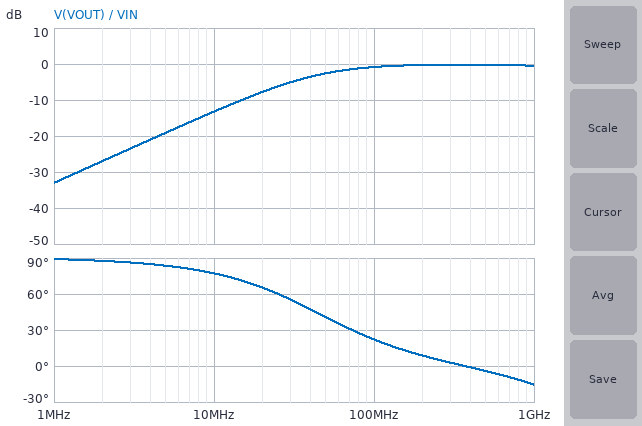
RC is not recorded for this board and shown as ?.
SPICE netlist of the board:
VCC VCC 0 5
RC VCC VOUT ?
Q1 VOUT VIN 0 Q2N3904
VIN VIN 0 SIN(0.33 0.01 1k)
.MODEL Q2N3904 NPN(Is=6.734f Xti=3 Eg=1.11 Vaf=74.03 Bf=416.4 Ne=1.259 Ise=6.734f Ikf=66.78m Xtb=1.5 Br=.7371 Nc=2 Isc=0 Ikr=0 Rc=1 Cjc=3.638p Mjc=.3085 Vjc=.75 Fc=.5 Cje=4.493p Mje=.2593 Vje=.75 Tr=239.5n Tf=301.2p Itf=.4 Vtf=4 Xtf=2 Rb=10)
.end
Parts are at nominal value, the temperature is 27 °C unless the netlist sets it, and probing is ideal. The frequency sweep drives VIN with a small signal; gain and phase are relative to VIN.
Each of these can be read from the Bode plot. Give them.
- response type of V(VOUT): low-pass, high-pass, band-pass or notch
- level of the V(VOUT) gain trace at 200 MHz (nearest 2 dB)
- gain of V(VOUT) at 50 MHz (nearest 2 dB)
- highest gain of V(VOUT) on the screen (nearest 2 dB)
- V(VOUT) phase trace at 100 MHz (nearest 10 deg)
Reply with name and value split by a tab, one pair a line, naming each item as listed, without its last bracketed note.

response type of V(VOUT): low-pass, high-pass, band-pass or notch	high-pass
level of the V(VOUT) gain trace at 200 MHz	0 dB
gain of V(VOUT) at 50 MHz	-2 dB
highest gain of V(VOUT) on the screen	0 dB
V(VOUT) phase trace at 100 MHz	20 deg
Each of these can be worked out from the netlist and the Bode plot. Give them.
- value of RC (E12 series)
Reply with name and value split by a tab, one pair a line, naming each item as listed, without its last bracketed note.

value of RC	1.8 kΩ
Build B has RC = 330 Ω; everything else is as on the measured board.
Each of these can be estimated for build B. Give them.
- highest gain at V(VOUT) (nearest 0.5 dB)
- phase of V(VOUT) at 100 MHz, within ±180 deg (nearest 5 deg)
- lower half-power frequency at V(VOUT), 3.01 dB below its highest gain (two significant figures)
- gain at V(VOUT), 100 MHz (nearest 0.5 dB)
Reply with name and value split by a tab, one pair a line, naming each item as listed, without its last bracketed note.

highest gain at V(VOUT)	-1.0 dB
phase of V(VOUT) at 100 MHz, within ±180 deg	65 deg
lower half-power frequency at V(VOUT), 3.01 dB below its highest gain	210 MHz
gain at V(VOUT), 100 MHz	-8.5 dB
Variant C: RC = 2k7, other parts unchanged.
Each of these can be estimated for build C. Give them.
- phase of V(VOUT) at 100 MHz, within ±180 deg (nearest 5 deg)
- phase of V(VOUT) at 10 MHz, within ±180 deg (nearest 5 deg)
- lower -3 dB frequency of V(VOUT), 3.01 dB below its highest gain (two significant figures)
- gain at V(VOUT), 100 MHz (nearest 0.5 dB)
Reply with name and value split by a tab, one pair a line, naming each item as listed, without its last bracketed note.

phase of V(VOUT) at 100 MHz, within ±180 deg	15 deg
phase of V(VOUT) at 10 MHz, within ±180 deg	70 deg
lower -3 dB frequency of V(VOUT), 3.01 dB below its highest gain	29 MHz
gain at V(VOUT), 100 MHz	-0.5 dB
